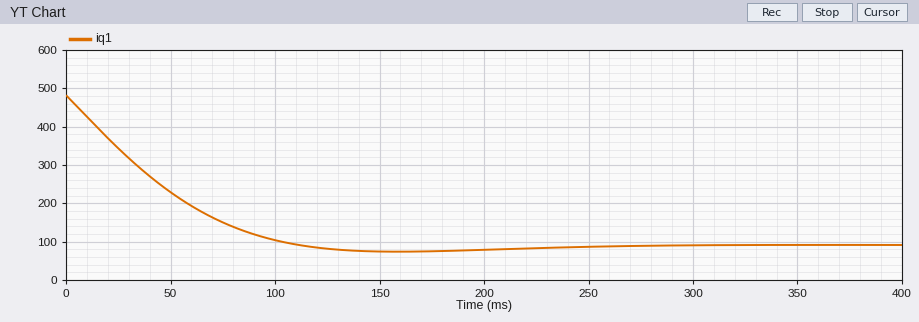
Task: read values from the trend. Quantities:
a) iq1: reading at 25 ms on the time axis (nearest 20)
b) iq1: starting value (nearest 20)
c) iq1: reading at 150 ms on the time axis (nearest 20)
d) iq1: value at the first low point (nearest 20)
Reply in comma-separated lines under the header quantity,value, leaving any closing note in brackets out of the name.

quantity,value
iq1: reading at 25 ms on the time axis,340
iq1: starting value,480
iq1: reading at 150 ms on the time axis,80
iq1: value at the first low point,80
